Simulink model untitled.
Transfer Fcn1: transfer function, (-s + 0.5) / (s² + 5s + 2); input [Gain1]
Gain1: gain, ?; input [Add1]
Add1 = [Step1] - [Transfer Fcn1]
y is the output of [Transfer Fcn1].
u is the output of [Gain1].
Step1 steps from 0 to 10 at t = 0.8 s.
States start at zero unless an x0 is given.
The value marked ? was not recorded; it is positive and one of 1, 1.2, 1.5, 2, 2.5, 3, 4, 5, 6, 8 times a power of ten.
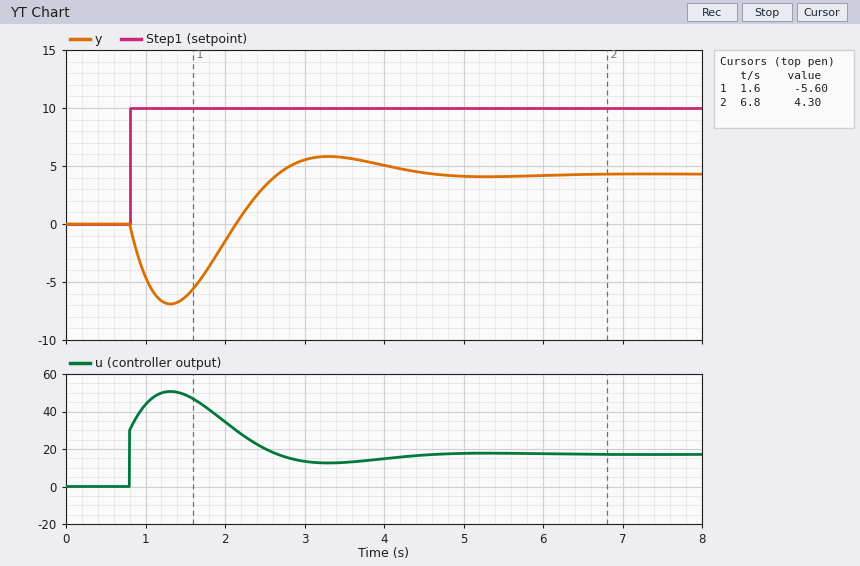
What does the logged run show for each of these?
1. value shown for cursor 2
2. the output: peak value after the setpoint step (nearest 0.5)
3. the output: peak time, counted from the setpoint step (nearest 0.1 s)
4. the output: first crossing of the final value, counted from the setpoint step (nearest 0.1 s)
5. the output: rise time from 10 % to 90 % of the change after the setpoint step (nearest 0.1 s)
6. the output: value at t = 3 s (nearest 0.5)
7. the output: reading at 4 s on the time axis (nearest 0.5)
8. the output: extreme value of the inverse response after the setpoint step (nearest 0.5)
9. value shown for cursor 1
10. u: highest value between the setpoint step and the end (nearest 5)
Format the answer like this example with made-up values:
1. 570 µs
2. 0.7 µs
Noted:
1. 4.30
2. 6.0
3. 2.5 s
4. 1.9 s
5. 0.4 s
6. 5.5
7. 5.0
8. -7.0
9. -5.60
10. 50
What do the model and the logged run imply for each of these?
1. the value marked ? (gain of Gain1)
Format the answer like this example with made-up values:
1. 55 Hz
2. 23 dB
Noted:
1. 3
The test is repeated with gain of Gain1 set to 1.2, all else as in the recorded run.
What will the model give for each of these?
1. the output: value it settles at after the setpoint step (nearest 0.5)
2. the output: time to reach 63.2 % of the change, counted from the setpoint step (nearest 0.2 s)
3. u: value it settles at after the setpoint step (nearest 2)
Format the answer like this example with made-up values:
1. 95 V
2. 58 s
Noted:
1. 2.5
2. 2.6 s
3. 10
